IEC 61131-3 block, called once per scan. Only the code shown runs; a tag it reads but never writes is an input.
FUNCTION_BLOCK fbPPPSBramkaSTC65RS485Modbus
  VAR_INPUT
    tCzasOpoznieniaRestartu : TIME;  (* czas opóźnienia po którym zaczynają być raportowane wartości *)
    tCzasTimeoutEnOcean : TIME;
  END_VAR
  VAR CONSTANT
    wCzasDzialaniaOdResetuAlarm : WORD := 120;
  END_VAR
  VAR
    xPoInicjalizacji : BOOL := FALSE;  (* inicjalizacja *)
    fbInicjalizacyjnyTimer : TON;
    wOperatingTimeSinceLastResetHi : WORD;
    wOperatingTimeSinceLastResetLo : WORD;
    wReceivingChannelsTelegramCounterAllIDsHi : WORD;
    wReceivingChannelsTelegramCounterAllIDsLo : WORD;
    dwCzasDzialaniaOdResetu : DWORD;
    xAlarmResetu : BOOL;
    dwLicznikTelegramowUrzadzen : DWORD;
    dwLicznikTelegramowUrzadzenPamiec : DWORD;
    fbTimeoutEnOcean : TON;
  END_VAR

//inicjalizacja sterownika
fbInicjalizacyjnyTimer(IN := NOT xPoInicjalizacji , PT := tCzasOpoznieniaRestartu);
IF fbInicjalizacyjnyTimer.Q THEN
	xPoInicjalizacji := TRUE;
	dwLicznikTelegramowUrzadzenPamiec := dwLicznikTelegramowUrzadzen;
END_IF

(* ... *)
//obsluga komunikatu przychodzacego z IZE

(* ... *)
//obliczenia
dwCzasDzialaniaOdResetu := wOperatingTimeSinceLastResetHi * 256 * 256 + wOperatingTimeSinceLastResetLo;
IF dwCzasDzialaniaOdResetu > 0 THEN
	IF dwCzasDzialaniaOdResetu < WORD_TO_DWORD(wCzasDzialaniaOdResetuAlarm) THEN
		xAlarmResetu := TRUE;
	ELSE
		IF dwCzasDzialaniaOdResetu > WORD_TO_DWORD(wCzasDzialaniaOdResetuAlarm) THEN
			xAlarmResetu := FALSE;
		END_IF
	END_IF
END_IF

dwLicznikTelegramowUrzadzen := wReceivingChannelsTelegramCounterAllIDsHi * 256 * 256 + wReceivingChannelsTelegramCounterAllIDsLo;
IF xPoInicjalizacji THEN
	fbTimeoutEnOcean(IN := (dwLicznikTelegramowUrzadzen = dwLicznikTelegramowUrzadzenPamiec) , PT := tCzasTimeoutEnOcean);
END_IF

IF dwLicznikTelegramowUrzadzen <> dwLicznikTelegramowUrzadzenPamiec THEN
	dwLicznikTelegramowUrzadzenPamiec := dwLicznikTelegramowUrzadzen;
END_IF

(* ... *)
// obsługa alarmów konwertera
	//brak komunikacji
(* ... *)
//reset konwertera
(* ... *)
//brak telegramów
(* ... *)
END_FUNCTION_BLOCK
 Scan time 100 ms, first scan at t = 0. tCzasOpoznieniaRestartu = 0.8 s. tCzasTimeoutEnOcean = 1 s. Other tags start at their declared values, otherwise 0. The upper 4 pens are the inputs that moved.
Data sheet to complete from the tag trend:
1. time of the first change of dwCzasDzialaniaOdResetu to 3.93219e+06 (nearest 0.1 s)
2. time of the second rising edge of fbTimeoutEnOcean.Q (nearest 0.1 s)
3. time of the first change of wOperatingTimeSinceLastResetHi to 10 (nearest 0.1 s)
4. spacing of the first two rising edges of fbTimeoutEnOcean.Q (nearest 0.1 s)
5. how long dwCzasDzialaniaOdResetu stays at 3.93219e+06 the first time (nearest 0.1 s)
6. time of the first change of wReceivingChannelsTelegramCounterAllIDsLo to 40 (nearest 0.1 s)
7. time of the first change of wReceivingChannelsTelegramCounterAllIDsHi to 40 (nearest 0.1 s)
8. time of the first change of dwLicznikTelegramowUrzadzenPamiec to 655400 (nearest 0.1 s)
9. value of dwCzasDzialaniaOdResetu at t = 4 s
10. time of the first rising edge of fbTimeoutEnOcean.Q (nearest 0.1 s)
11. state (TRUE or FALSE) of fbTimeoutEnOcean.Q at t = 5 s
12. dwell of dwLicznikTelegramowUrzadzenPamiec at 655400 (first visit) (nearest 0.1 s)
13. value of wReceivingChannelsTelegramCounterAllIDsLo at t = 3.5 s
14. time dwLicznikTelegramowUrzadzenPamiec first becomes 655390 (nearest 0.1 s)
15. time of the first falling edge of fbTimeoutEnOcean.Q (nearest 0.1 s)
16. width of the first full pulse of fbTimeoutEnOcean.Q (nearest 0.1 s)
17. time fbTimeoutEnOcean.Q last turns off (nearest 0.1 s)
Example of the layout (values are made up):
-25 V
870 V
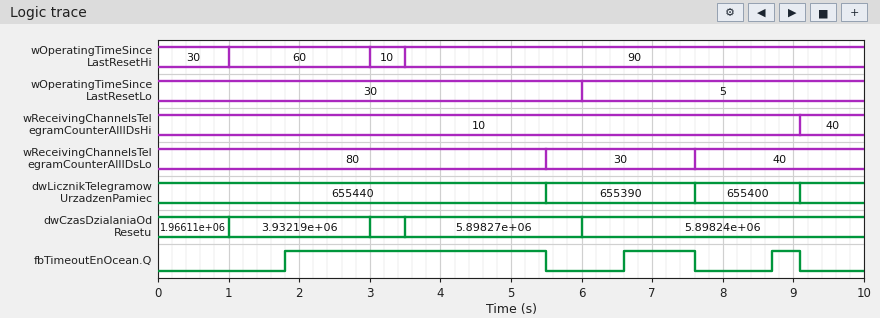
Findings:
1.0 s
6.6 s
3.0 s
4.8 s
2.0 s
7.6 s
9.1 s
7.6 s
5.89827e+06
1.8 s
TRUE
1.5 s
80
5.5 s
5.5 s
3.7 s
9.1 s
